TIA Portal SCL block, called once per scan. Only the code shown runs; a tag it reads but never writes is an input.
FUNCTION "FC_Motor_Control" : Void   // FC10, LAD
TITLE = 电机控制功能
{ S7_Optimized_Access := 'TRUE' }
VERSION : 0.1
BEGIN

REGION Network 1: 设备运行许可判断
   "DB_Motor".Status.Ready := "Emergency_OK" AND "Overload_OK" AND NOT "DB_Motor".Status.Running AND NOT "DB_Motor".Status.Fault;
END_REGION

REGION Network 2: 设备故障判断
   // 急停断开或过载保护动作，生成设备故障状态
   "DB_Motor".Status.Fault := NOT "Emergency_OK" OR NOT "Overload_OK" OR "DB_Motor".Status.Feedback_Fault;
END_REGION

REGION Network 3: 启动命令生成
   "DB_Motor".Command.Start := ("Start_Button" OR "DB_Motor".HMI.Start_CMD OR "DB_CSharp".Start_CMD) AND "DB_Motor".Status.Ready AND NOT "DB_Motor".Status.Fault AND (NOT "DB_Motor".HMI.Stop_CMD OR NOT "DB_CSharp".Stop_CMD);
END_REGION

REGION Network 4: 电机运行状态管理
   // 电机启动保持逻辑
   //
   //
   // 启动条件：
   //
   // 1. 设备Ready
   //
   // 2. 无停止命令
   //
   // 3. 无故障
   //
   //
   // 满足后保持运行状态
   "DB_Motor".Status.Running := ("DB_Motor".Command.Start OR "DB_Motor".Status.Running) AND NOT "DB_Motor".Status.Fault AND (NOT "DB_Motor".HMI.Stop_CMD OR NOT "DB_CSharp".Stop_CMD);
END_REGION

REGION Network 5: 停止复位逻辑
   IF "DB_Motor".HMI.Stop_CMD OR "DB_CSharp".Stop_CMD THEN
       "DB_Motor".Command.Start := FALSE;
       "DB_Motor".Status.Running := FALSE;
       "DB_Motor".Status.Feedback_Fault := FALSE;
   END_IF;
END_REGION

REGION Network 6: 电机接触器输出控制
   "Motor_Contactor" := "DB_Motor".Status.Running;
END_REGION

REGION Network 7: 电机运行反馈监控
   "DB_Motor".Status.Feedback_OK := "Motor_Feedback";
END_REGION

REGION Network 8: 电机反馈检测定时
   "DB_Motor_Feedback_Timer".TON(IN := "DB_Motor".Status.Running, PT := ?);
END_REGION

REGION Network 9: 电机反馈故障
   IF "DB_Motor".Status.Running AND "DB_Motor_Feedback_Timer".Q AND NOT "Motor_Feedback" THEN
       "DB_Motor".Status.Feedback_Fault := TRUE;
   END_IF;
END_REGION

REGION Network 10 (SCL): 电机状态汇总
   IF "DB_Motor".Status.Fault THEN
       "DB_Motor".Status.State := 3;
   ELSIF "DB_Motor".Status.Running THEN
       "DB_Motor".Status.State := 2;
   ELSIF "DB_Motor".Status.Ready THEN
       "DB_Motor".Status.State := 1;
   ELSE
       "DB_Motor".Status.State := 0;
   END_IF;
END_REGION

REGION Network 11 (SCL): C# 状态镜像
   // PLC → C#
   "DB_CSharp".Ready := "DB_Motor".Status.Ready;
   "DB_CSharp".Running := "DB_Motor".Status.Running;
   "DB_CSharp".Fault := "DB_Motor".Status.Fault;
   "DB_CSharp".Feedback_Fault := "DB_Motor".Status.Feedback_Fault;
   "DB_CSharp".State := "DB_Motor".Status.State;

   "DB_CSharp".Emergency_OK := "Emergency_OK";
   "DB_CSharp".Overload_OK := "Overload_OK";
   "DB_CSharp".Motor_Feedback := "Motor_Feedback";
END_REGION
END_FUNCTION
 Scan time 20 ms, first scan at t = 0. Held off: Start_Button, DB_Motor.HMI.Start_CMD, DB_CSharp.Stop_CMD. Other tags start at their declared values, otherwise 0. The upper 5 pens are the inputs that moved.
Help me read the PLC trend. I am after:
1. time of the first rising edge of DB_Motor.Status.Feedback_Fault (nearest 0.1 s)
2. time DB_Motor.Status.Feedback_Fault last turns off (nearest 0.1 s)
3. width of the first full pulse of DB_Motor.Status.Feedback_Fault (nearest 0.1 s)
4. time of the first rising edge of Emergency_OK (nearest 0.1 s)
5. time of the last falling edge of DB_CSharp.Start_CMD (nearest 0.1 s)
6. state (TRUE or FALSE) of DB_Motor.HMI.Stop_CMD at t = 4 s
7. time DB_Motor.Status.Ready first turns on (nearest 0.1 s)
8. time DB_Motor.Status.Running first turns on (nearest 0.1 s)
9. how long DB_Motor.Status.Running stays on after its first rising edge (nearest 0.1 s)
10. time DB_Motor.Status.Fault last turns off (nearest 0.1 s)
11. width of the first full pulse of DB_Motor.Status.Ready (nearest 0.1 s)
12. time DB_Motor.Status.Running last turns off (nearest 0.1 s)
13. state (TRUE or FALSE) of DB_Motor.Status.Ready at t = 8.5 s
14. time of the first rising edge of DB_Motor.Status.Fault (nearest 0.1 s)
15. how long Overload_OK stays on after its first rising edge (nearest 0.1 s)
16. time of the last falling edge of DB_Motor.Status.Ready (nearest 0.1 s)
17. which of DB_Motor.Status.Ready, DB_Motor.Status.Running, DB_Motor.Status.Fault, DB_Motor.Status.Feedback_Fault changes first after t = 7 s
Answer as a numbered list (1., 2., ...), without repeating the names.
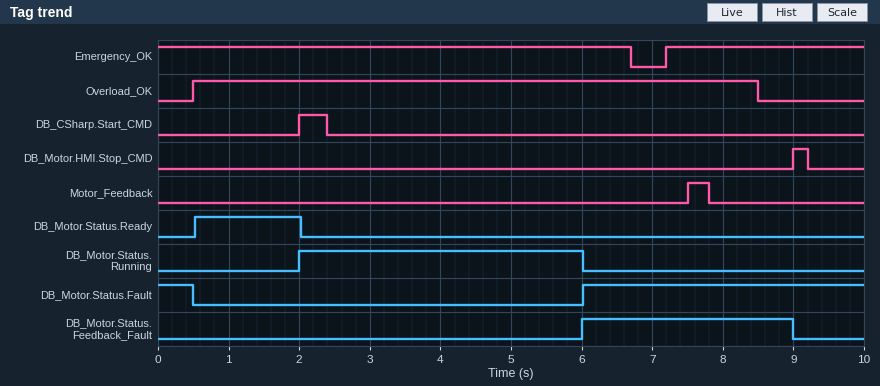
1. 6.0 s
2. 9.0 s
3. 3.0 s
4. 7.2 s
5. 2.4 s
6. FALSE
7. 0.5 s
8. 2.0 s
9. 4.0 s
10. 0.5 s
11. 1.5 s
12. 6.0 s
13. FALSE
14. 6.0 s
15. 8.0 s
16. 2.0 s
17. DB_Motor.Status.Feedback_Fault
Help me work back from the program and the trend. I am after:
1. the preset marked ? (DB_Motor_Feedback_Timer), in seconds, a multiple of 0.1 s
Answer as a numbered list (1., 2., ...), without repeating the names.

1. 4.0 s
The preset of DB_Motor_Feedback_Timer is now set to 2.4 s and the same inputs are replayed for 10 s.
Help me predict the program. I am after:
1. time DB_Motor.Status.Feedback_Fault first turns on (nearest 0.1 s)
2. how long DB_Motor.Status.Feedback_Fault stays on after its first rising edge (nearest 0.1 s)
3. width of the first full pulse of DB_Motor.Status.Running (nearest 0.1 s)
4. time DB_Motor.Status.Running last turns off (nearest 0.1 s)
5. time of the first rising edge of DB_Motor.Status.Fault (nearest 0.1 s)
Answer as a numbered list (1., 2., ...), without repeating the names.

1. 4.4 s
2. 4.6 s
3. 2.4 s
4. 4.4 s
5. 4.4 s
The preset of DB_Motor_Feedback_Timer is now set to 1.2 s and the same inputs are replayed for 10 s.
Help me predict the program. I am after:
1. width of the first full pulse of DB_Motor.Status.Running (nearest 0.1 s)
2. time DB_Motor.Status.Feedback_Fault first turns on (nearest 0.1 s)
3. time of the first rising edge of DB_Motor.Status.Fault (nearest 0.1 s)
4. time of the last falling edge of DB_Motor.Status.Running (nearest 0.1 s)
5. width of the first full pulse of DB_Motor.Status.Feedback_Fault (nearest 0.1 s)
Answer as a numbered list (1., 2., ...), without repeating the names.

1. 1.2 s
2. 3.2 s
3. 3.2 s
4. 3.2 s
5. 5.8 s
